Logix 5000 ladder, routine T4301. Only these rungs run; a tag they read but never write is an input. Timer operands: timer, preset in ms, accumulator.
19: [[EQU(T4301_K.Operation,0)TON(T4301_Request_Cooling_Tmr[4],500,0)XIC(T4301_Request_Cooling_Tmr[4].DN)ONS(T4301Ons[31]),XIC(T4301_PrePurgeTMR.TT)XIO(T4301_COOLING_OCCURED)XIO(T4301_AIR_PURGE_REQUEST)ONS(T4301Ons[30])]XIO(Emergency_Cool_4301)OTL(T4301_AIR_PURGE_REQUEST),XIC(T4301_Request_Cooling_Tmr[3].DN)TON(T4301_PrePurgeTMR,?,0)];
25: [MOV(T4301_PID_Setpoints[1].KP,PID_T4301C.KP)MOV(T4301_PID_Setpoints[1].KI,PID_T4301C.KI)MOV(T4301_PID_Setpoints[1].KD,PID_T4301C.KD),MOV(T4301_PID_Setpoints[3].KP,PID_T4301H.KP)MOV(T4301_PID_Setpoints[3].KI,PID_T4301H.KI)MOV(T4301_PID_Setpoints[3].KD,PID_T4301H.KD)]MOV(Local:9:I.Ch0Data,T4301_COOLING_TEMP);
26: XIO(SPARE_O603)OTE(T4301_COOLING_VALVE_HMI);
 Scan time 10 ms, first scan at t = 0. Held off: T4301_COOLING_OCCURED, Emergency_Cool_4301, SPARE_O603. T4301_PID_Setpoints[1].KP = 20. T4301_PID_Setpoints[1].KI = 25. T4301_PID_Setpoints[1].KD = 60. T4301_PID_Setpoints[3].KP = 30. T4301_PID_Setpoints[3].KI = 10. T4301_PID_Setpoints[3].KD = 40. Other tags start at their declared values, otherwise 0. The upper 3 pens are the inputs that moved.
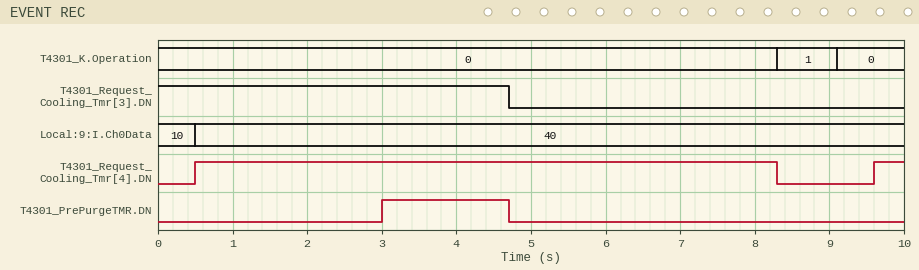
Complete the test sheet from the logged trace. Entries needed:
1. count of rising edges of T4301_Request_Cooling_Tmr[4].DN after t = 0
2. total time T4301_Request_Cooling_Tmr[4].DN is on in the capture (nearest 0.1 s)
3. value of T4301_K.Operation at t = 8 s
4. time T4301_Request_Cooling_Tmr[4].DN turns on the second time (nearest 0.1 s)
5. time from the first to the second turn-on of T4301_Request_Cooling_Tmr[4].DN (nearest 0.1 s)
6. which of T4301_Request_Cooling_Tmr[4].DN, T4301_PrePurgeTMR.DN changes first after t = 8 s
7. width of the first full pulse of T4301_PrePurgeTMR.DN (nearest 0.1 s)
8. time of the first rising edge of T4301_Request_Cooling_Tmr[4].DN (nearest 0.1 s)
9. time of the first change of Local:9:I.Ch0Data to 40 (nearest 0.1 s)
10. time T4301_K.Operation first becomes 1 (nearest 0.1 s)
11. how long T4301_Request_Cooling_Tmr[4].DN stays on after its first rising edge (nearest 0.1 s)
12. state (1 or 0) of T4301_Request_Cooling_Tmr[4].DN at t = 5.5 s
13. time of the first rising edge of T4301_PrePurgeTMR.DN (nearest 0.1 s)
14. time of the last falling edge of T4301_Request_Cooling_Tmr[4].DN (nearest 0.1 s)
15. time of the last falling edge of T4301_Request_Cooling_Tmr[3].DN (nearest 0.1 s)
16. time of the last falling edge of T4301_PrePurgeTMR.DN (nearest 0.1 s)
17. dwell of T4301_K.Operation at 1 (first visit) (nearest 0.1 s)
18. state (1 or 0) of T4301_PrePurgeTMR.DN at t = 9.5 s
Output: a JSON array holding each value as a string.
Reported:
["2", "8.2 s", "0", "9.6 s", "9.1 s", "T4301_Request_Cooling_Tmr[4].DN", "1.7 s", "0.5 s", "0.5 s", "8.3 s", "7.8 s", "1", "3.0 s", "8.3 s", "4.7 s", "4.7 s", "0.8 s", "0"]
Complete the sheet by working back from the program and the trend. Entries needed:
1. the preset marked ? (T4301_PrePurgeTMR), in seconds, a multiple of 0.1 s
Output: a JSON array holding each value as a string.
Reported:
["3.0 s"]
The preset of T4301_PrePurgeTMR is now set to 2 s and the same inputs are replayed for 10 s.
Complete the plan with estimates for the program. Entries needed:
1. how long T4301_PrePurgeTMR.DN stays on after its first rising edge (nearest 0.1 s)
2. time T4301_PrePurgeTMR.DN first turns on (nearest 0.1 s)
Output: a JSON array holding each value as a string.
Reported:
["2.7 s", "2.0 s"]
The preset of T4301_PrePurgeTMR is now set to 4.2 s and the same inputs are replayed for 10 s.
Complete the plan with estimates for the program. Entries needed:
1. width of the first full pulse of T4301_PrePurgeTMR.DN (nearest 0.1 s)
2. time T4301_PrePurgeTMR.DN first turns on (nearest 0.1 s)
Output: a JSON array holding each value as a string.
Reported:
["0.5 s", "4.2 s"]
